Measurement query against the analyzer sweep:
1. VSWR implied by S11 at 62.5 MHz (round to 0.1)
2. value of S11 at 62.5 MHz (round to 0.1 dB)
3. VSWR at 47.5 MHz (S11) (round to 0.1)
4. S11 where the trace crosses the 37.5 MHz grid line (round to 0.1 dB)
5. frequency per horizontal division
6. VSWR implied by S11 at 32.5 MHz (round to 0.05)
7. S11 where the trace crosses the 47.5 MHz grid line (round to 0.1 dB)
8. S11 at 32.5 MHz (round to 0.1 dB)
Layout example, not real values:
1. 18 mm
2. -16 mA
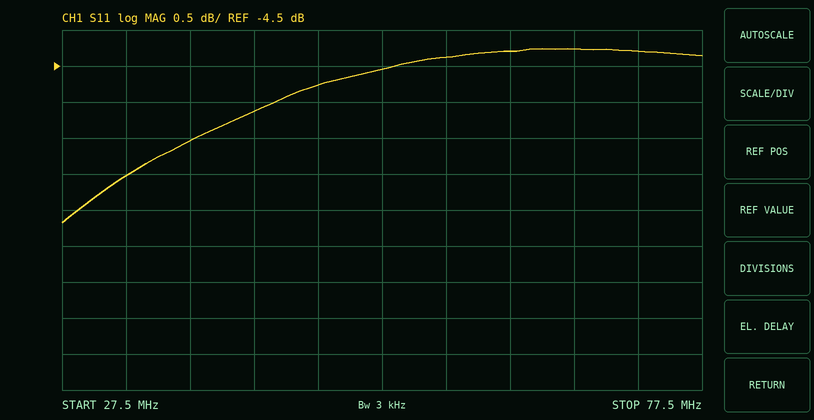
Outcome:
1. 4.1
2. -4.3 dB
3. 3.7
4. -5.5 dB
5. 5 MHz
6. 3.00
7. -4.8 dB
8. -6.0 dB
